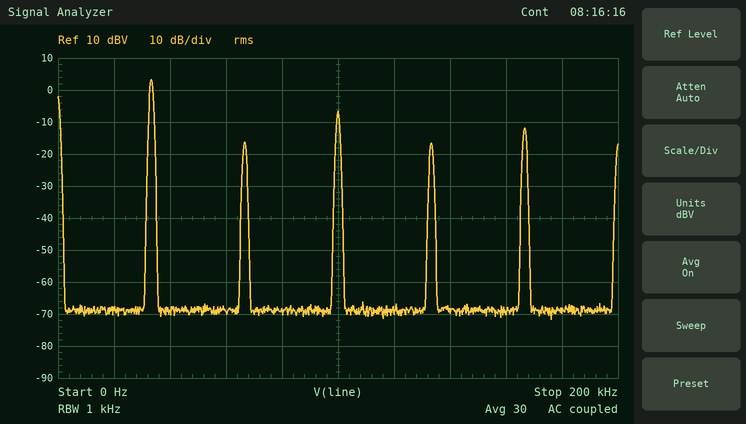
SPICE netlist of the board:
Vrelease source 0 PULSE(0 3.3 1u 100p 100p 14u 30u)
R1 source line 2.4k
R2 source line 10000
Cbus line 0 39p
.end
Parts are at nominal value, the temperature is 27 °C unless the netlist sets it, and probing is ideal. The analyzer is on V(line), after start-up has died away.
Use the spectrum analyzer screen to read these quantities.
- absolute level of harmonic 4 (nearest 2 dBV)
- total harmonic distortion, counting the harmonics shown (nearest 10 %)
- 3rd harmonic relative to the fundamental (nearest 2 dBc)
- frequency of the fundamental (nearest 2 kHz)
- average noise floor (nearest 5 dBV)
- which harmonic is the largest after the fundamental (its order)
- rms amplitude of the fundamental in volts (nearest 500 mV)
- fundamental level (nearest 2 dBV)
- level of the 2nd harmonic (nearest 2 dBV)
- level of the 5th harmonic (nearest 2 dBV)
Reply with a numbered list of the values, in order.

1. -16 dBV
2. 40 %
3. -10 dBc
4. 34 kHz
5. -70 dBV
6. 3
7. 1.5 V
8. 4 dBV
9. -16 dBV
10. -12 dBV
